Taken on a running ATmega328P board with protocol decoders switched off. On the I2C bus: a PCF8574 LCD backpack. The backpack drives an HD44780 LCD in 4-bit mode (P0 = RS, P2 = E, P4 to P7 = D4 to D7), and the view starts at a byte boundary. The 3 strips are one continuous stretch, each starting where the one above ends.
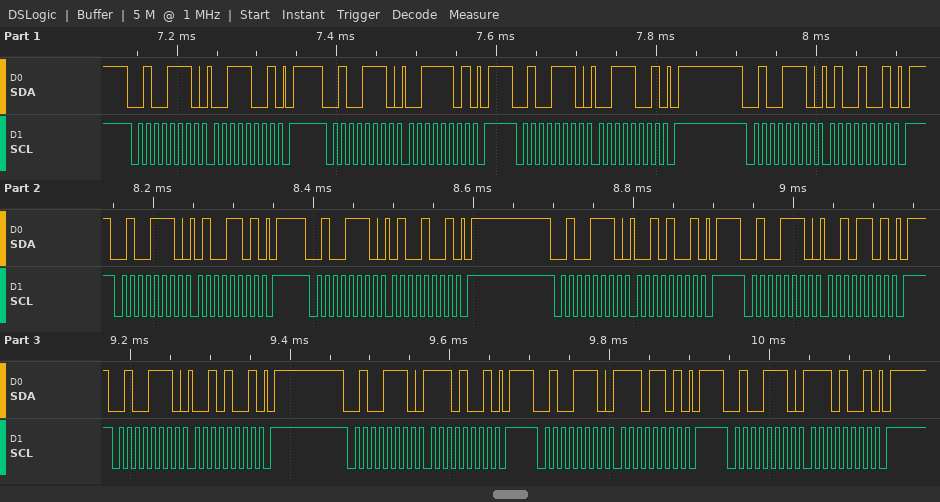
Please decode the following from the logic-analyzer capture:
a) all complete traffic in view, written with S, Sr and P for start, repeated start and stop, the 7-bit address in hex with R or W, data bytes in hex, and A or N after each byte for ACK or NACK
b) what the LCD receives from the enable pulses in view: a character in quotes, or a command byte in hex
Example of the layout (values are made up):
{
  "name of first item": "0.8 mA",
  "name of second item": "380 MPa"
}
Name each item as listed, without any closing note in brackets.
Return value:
{
  "all complete traffic in view, written with S, Sr and P for start, repeated start and stop, the 7-bit address in hex with R or W, data bytes in hex, and A or N after each byte for ACK or NACK": "S 27W A 39 A P S 27W A 3D A P S 27W A 39 A P S 27W A 49 A P S 27W A 4D A P S 27W A 49 A P S 27W A 29 A P S 27W A 2D A P S 27W A 29 A P S 27W A E9 A P S 27W A ED A P S 27W A E9 A P",
  "what the LCD receives from the enable pulses in view: a character in quotes, or a command byte in hex": "'4' '.'"
}
